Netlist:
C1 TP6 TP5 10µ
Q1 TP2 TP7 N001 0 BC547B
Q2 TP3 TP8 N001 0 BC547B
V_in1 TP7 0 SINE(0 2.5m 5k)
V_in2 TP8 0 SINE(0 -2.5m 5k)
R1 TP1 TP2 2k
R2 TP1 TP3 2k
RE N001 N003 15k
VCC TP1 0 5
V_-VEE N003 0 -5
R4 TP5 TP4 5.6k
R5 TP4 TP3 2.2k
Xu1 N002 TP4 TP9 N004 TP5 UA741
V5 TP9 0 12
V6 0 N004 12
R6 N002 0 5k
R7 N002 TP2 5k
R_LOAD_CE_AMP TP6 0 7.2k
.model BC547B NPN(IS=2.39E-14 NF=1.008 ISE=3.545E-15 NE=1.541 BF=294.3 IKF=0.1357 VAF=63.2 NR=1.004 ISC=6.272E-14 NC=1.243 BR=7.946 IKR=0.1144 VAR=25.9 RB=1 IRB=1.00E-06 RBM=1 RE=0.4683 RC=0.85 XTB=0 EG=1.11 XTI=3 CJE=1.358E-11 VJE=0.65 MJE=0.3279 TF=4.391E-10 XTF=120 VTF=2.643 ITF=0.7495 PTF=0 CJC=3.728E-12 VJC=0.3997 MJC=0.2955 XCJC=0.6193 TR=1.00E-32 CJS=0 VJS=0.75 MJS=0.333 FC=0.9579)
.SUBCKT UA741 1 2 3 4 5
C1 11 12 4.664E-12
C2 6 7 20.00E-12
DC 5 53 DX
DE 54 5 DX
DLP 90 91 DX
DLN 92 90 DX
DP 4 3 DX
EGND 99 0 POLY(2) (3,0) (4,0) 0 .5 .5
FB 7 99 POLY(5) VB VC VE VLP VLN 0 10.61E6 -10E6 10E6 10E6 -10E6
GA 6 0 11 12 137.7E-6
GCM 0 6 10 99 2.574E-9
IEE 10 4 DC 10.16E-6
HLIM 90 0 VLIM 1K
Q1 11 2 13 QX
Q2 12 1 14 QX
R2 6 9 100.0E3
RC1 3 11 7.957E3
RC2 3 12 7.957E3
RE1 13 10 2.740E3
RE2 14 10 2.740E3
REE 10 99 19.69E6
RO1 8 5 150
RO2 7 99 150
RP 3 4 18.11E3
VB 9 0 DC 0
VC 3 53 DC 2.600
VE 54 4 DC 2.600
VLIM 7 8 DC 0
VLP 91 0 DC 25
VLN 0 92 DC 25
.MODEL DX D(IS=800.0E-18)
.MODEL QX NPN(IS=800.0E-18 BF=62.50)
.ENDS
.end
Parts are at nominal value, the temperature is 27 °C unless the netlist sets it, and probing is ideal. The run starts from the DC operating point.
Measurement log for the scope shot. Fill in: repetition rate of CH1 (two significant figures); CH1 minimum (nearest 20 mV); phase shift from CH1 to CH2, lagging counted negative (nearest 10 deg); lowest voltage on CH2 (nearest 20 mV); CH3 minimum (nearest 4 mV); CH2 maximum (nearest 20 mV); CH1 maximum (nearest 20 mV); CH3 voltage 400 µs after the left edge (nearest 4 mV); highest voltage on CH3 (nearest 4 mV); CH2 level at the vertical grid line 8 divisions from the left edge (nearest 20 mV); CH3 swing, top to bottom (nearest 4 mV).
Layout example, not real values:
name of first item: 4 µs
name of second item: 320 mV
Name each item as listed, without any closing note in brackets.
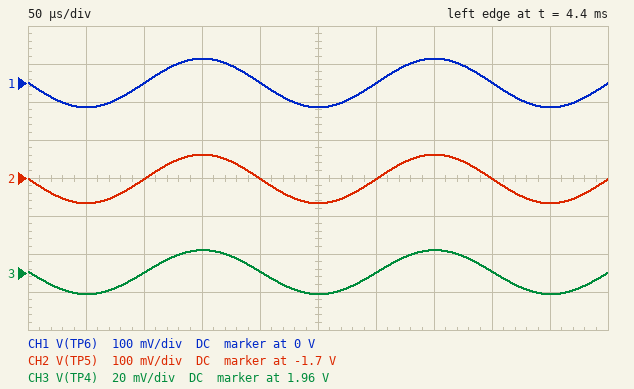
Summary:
repetition rate of CH1: 5.0 kHz
CH1 minimum: -60 mV
phase shift from CH1 to CH2, lagging counted negative: 0 deg
lowest voltage on CH2: -1.76 V
CH3 minimum: 1.948 V
CH2 maximum: -1.64 V
CH1 maximum: 60 mV
CH3 voltage 400 µs after the left edge: 1.960 V
highest voltage on CH3: 1.972 V
CH2 level at the vertical grid line 8 divisions from the left edge: -1.70 V
CH3 swing, top to bottom: 24 mV
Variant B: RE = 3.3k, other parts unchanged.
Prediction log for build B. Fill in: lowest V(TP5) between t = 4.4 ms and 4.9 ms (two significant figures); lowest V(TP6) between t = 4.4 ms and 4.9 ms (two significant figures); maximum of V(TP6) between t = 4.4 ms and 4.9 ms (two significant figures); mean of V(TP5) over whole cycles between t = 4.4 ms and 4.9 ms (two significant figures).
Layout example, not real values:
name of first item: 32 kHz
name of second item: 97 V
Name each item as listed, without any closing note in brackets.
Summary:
lowest V(TP5) between t = 4.4 ms and 4.9 ms: -1.6 V
lowest V(TP6) between t = 4.4 ms and 4.9 ms: -280 mV
maximum of V(TP6) between t = 4.4 ms and 4.9 ms: 280 mV
mean of V(TP5) over whole cycles between t = 4.4 ms and 4.9 ms: -1.3 V
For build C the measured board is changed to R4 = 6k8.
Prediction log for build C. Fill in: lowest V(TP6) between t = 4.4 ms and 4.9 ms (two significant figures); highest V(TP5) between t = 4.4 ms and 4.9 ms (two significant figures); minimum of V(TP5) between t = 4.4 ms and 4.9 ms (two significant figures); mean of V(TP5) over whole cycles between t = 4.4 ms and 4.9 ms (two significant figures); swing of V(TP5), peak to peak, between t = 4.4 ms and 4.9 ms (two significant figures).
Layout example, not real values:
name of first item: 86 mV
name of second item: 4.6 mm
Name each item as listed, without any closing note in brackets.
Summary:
lowest V(TP6) between t = 4.4 ms and 4.9 ms: -75 mV
highest V(TP5) between t = 4.4 ms and 4.9 ms: -2.4 V
minimum of V(TP5) between t = 4.4 ms and 4.9 ms: -2.6 V
mean of V(TP5) over whole cycles between t = 4.4 ms and 4.9 ms: -2.5 V
swing of V(TP5), peak to peak, between t = 4.4 ms and 4.9 ms: 150 mV
